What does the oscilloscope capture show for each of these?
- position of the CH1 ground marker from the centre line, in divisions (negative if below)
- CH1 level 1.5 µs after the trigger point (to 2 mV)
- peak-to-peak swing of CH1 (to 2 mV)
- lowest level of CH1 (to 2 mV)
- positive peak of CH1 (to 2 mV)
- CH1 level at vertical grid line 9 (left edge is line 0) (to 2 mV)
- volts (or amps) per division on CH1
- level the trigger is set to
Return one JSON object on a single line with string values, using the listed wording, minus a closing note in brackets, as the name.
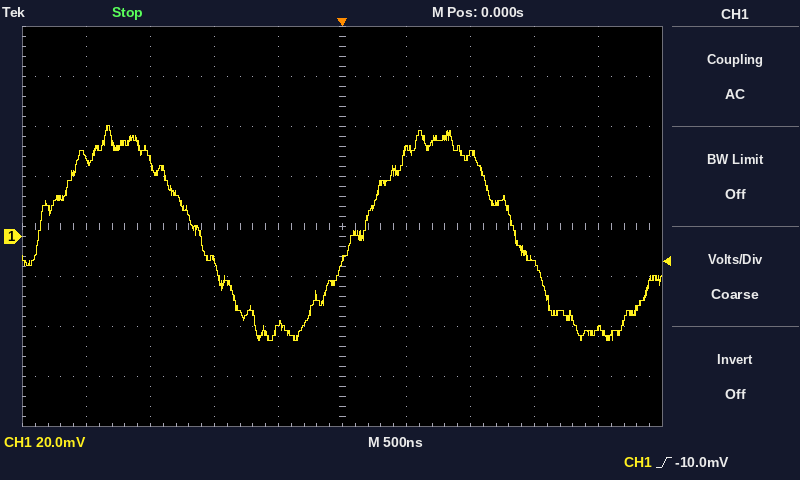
{"position of the CH1 ground marker from the centre line, in divisions": "-0.2 div", "CH1 level 1.5 µs after the trigger point": "-10 mV", "peak-to-peak swing of CH1": "86 mV", "lowest level of CH1": "-42 mV", "positive peak of CH1": "44 mV", "CH1 level at vertical grid line 9 (left edge is line 0)": "-36 mV", "volts (or amps) per division on CH1": "20 mV", "level the trigger is set to": "-10.0 mV"}
